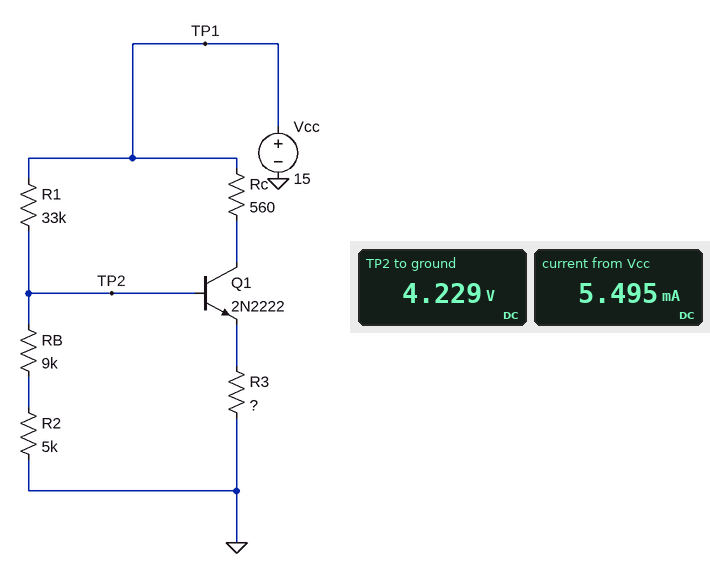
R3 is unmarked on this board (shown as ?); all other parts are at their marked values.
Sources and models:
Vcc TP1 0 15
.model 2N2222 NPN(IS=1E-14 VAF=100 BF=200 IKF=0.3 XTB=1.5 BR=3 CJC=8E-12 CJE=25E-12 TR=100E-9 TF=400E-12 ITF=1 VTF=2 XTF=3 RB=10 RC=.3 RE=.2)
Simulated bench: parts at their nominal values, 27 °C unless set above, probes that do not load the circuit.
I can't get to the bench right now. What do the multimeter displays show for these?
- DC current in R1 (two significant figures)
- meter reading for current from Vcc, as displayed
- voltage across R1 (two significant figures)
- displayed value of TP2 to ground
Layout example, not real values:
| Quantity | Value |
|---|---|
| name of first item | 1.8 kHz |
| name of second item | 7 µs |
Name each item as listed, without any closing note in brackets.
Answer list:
| Quantity | Value |
|---|---|
| DC current in R1 | 330 µA |
| meter reading for current from Vcc, as displayed | 5.495 mA |
| voltage across R1 | 11 V |
| displayed value of TP2 to ground | 4.229 V |
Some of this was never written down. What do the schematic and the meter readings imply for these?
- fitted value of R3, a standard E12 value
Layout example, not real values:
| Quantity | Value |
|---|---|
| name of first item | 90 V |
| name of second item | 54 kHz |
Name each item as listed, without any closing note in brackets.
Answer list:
| Quantity | Value |
|---|---|
| fitted value of R3, a standard E12 value | 680 Ω |
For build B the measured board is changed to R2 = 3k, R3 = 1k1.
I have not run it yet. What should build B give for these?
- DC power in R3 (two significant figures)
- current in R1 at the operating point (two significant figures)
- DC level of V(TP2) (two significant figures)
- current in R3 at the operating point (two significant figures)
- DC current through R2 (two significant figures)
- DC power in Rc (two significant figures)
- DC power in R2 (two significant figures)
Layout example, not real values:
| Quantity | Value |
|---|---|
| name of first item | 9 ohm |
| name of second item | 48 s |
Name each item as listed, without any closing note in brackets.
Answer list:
| Quantity | Value |
|---|---|
| DC power in R3 | 9.3 mW |
| current in R1 at the operating point | 340 µA |
| DC level of V(TP2) | 3.9 V |
| current in R3 at the operating point | 2.9 mA |
| DC current through R2 | 320 µA |
| DC power in Rc | 4.7 mW |
| DC power in R2 | 310 µW |
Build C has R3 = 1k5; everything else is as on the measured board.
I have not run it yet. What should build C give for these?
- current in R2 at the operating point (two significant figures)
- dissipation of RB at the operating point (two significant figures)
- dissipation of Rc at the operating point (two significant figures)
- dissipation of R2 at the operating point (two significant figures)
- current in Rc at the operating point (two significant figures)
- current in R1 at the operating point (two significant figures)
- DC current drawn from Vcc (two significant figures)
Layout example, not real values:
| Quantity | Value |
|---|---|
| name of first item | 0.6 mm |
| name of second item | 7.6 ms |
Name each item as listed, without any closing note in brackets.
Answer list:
| Quantity | Value |
|---|---|
| current in R2 at the operating point | 310 µA |
| dissipation of RB at the operating point | 870 µW |
| dissipation of Rc at the operating point | 3.3 mW |
| dissipation of R2 at the operating point | 480 µW |
| current in Rc at the operating point | 2.4 mA |
| current in R1 at the operating point | 320 µA |
| DC current drawn from Vcc | 2.8 mA |
